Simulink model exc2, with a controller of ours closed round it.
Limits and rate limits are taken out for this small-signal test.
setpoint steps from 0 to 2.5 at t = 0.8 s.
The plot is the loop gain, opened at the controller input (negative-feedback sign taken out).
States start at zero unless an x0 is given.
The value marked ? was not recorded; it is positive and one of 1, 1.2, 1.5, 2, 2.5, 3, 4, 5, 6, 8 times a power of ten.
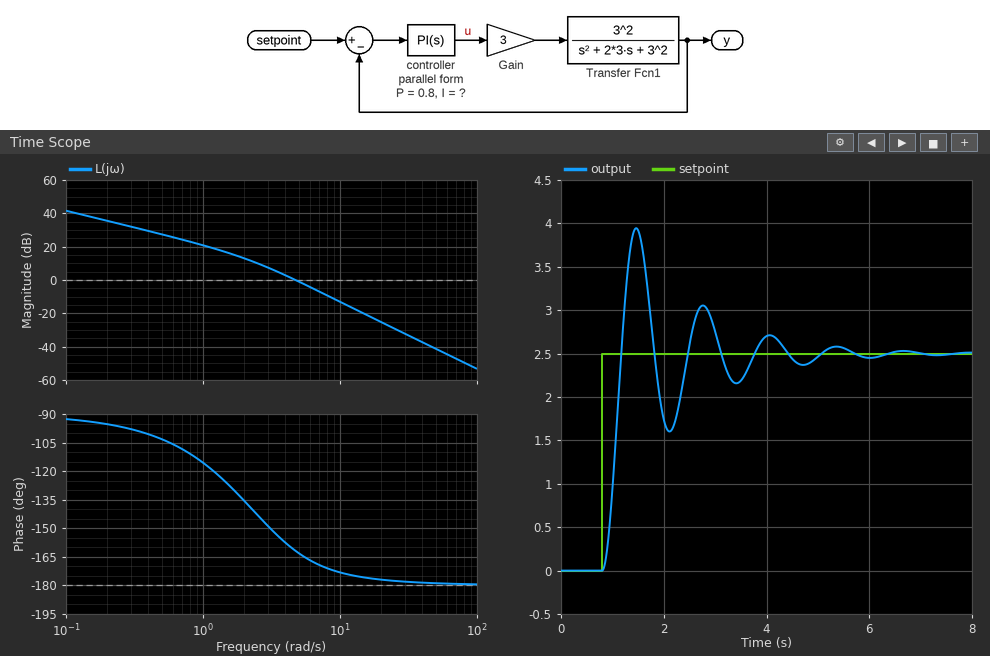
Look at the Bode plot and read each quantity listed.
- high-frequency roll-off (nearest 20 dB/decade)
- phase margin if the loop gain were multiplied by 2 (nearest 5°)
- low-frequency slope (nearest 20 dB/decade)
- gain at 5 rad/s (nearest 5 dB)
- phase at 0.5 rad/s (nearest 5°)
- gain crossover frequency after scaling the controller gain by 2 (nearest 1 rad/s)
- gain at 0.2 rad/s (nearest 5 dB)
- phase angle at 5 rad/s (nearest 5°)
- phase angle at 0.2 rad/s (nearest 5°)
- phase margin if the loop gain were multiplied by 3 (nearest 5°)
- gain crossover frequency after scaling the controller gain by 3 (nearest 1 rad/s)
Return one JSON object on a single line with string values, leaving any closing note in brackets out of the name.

{"high-frequency roll-off": "-40 dB/decade", "phase margin if the loop gain were multiplied by 2": "10°", "low-frequency slope": "-20 dB/decade", "gain at 5 rad/s": "0 dB", "phase at 0.5 rad/s": "-105°", "gain crossover frequency after scaling the controller gain by 2": "7 rad/s", "gain at 0.2 rad/s": "35 dB", "phase angle at 5 rad/s": "-165°", "phase angle at 0.2 rad/s": "-95°", "phase margin if the loop gain were multiplied by 3": "10°", "gain crossover frequency after scaling the controller gain by 3": "8 rad/s"}
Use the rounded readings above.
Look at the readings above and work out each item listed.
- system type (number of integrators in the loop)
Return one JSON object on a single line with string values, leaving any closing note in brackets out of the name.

{"system type": "1"}
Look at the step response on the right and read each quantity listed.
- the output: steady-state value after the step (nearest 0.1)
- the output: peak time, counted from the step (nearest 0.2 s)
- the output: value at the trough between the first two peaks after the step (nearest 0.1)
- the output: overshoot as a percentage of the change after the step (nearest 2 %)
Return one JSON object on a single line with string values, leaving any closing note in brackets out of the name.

{"the output: steady-state value after the step": "2.5", "the output: peak time, counted from the step": "0.6 s", "the output: value at the trough between the first two peaks after the step": "1.6", "the output: overshoot as a percentage of the change after the step": "58 %"}
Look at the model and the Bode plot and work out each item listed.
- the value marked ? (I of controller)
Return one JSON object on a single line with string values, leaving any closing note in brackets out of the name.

{"the value marked ?": "4"}
